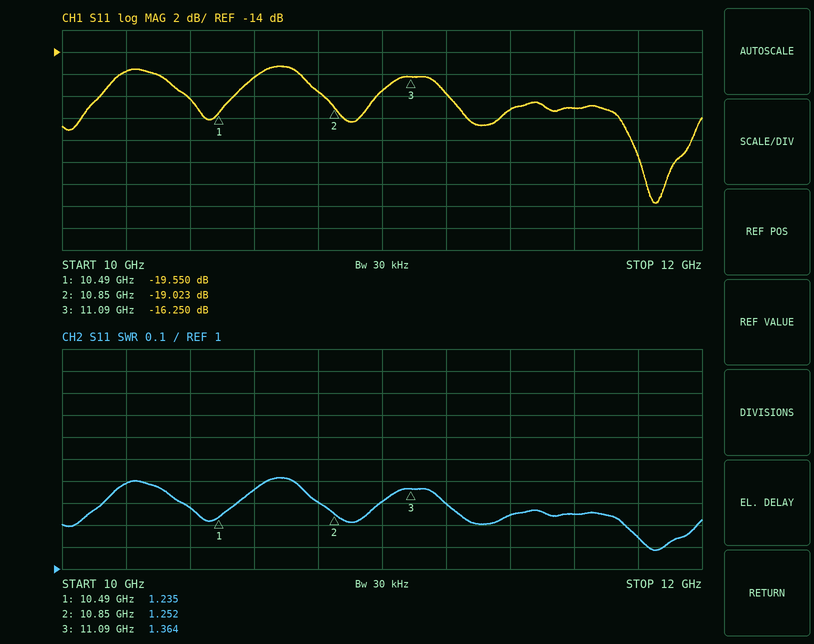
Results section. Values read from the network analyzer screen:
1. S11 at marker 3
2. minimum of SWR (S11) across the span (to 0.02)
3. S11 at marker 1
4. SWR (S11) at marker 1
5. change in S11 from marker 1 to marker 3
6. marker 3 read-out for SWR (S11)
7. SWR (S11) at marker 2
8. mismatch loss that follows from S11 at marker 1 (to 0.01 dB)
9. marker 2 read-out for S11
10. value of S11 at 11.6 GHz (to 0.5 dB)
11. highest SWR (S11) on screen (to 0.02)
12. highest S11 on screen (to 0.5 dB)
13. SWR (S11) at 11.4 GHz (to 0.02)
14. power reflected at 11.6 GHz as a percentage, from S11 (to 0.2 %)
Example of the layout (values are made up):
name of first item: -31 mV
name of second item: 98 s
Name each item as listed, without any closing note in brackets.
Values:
S11 at marker 3: -16.250 dB
minimum of SWR (S11) across the span: 1.08
S11 at marker 1: -19.550 dB
SWR (S11) at marker 1: 1.235
change in S11 from marker 1 to marker 3: 3.300 dB
marker 3 read-out for SWR: 1.364
SWR (S11) at marker 2: 1.252
mismatch loss that follows from S11 at marker 1: 0.05 dB
marker 2 read-out for S11: -19.023 dB
value of S11 at 11.6 GHz: -19.0 dB
highest SWR (S11) on screen: 1.42
highest S11 on screen: -15.5 dB
SWR (S11) at 11.4 GHz: 1.24
power reflected at 11.6 GHz as a percentage, from S11: 1.2 %
